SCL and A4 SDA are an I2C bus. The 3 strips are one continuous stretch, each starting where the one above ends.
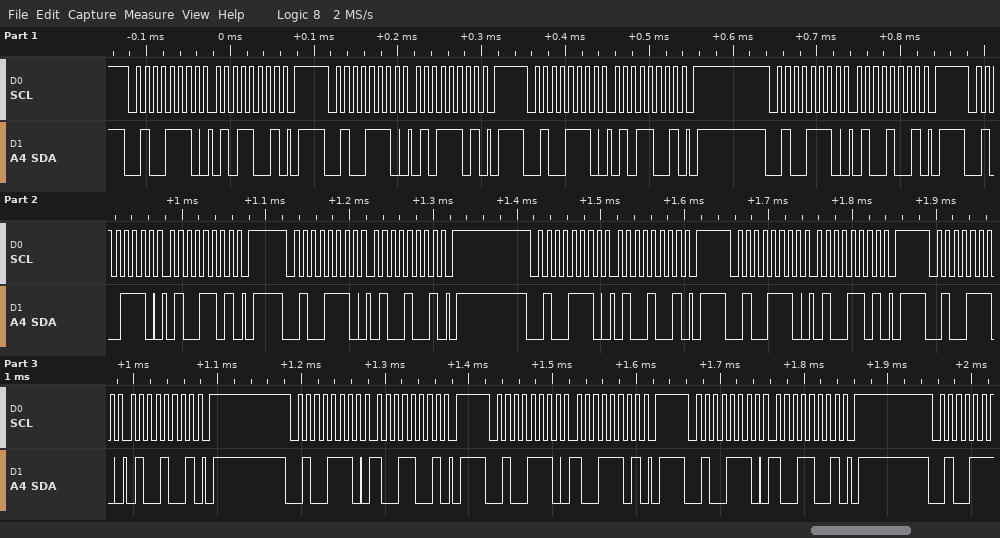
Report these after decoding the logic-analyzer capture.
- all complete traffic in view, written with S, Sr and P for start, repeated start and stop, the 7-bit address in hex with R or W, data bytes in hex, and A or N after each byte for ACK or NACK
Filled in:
S 27W A 59 A P S 27W A 5D A P S 27W A 59 A P S 27W A 49 A P S 27W A 4D A P S 27W A 49 A P S 27W A 49 A P S 27W A 4D A P S 27W A 49 A P S 27W A 99 A P S 27W A 9D A P S 27W A 99 A P
